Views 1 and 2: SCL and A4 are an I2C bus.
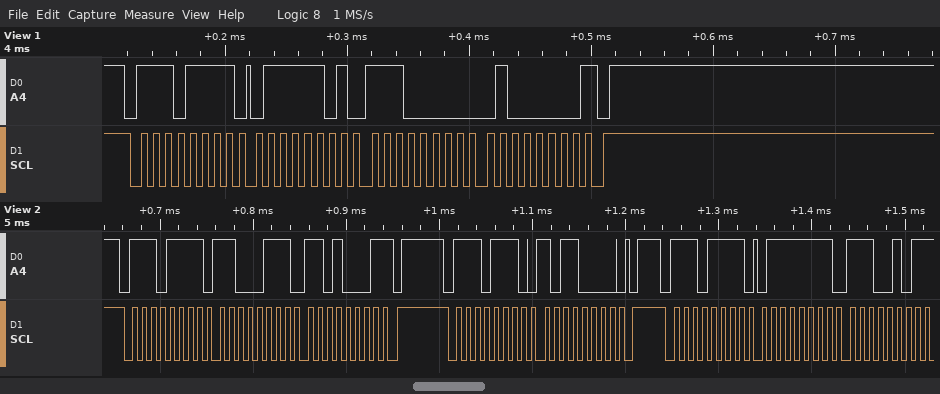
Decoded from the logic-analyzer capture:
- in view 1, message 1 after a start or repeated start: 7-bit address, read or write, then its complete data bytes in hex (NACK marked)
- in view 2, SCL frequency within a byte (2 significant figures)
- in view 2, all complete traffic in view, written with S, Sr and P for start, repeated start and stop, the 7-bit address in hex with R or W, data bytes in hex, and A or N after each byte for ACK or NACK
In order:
0x77 read: 7D E0 40 NACK
100 kHz
S 77R A C7 A D1 N P S 77W A B0 A P S 77R A 7F A E5 N
